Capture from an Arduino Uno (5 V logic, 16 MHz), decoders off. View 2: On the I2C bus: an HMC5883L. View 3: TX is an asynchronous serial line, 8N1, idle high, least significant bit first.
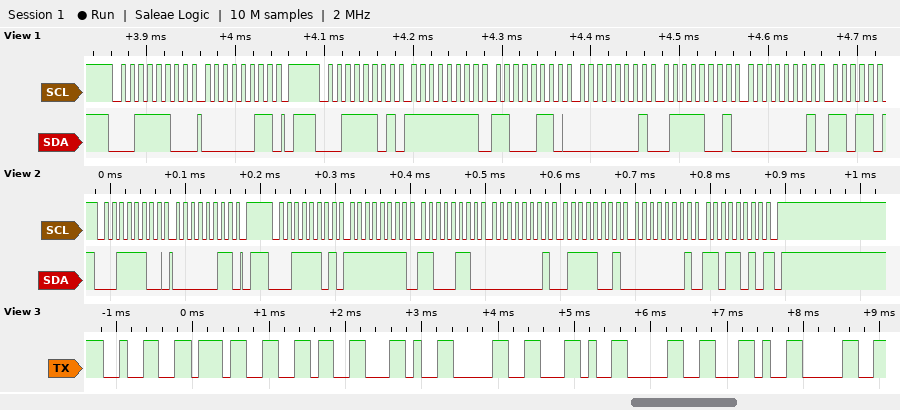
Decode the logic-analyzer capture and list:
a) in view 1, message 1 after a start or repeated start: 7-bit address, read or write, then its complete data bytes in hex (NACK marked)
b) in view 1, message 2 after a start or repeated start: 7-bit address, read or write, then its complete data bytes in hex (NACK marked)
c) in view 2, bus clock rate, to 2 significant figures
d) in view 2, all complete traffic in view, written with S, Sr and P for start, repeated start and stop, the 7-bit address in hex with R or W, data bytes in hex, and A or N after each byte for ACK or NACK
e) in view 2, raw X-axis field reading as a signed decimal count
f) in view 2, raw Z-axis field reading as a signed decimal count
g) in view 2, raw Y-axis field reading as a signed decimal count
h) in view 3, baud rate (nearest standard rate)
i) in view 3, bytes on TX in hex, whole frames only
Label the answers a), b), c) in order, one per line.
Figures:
a) 0x1E write: 03
b) 0x1E read: FF C6 01 79 01
c) 100 kHz
d) S 1EW A 03 A P S 1ER A FF A C6 A 01 A 79 A 01 A DA N P
e) -58
f) 377
g) 474
h) 9600 baud
i) 32 37 36 2C 30 2C 30 2C 30
